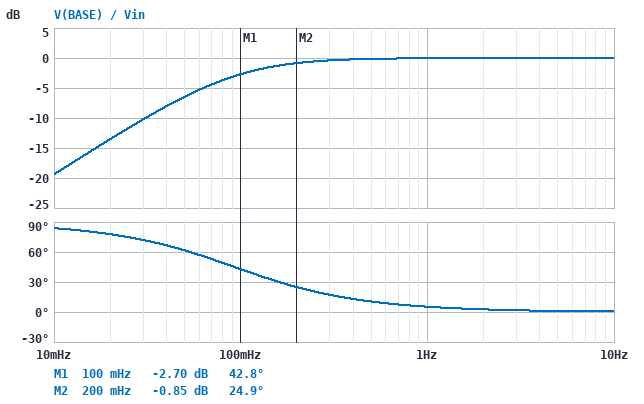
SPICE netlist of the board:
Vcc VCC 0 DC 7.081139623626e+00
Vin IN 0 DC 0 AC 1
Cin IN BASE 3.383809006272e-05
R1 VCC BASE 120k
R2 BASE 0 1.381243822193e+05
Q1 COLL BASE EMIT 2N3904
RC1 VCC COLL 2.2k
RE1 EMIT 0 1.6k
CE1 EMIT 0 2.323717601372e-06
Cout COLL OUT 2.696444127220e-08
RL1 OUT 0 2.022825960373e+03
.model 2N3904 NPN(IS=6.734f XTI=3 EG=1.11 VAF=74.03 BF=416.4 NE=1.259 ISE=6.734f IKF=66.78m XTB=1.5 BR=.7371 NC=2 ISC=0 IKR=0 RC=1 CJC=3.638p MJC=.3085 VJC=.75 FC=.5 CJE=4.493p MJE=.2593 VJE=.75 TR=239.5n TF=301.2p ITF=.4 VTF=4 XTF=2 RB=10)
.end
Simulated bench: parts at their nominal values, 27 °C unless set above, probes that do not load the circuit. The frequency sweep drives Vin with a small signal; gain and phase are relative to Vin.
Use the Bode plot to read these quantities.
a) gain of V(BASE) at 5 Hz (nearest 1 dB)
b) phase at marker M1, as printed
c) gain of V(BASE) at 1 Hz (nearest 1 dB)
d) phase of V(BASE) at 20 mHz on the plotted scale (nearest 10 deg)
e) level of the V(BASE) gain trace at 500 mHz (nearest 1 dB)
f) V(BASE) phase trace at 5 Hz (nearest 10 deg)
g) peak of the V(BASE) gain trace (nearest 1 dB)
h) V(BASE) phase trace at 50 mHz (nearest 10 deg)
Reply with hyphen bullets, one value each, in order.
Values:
- 0 dB
- 42.8 deg
- 0 dB
- 80 deg
- 0 dB
- 0 deg
- 0 dB
- 60 deg
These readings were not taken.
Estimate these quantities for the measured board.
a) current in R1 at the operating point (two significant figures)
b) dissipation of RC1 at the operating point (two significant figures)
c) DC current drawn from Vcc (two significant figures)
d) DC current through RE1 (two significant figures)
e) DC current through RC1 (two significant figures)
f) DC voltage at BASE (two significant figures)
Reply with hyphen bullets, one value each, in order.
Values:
- 33 µA
- 5.0 mW
- 1.5 mA
- 1.5 mA
- 1.5 mA
- 3.1 V
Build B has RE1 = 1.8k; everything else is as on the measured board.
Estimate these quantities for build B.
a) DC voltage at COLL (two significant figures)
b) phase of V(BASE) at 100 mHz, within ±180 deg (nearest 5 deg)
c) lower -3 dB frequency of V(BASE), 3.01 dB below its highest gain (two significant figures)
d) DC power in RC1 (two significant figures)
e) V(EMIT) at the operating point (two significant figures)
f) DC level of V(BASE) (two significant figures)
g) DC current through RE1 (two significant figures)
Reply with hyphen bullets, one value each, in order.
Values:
- 4.1 V
- 40 deg
- 91 mHz
- 4.1 mW
- 2.5 V
- 3.2 V
- 1.4 mA
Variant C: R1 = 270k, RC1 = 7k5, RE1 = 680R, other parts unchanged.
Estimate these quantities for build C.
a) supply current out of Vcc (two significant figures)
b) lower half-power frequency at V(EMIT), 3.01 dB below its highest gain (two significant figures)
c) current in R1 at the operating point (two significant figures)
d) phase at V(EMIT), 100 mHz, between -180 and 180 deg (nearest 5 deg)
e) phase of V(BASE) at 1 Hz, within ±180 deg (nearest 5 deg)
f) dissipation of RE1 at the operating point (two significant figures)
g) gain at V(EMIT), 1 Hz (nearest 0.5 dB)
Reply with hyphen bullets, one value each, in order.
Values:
- 870 µA
- 4.3 Hz
- 22 µA
- 90 deg
- 75 deg
- 500 µW
- -14.0 dB
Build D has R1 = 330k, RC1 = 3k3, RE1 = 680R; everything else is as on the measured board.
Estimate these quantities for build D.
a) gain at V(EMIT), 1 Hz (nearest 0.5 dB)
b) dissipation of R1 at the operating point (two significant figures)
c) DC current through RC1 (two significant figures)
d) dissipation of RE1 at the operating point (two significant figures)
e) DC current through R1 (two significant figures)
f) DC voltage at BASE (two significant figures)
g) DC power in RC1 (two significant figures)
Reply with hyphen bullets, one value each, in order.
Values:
- -0.5 dB
- 99 µW
- 1.0 mA
- 720 µW
- 17 µA
- 1.4 V
- 3.4 mW
